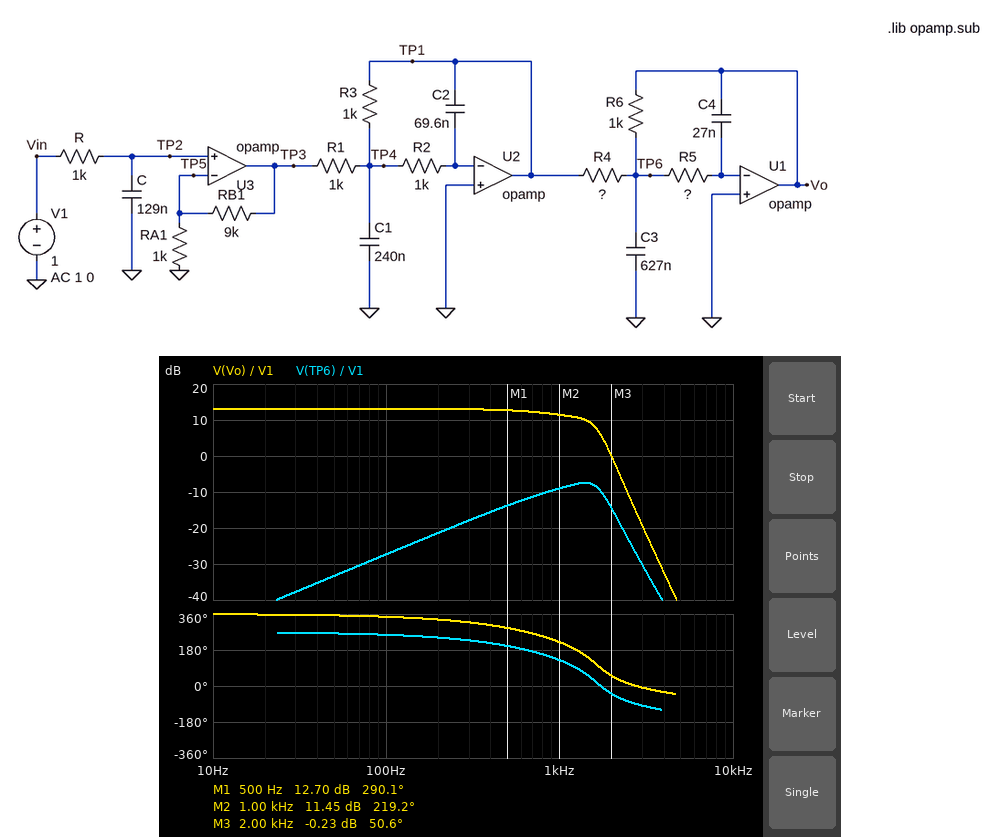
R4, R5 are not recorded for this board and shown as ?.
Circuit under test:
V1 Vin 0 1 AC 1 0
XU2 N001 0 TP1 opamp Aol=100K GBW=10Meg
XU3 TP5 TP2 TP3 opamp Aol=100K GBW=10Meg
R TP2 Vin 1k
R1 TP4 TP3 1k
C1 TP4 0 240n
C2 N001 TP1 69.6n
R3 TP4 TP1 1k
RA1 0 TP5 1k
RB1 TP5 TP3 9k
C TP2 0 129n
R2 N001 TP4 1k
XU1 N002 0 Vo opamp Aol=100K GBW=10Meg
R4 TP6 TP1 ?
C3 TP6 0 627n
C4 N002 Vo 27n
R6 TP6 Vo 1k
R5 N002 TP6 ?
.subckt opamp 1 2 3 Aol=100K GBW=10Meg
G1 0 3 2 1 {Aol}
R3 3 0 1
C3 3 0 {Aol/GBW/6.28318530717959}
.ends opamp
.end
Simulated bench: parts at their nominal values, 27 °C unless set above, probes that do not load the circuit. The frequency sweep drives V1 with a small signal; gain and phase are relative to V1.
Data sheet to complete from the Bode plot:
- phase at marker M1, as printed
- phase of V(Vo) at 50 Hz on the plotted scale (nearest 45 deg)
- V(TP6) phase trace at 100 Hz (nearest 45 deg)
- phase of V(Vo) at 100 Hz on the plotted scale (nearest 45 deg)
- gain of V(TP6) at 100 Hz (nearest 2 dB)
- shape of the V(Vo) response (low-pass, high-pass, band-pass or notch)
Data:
290.1 deg
360 deg
270 deg
360 deg
-28 dB
low-pass
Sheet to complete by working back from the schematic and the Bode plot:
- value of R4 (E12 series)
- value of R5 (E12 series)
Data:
2.2 kΩ
560 Ω
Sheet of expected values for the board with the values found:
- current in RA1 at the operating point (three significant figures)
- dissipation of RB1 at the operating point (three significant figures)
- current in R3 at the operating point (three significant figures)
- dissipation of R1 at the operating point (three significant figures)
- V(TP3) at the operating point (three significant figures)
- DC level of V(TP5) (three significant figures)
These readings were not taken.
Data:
1.00 mA
9.00 mW
10.0 mA
100 mW
10.0 V
1.00 V
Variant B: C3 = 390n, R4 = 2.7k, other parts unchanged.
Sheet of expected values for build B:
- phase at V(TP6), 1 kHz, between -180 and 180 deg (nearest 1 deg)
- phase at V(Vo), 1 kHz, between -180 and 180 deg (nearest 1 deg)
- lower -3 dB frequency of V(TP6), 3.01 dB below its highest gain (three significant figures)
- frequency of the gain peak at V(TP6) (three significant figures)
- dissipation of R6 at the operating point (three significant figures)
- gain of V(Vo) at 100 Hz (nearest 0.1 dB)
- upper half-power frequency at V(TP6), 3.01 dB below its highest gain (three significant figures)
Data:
134 deg
-136 deg
579 Hz
1.32 kHz
13.7 mW
11.3 dB
2.08 kHz
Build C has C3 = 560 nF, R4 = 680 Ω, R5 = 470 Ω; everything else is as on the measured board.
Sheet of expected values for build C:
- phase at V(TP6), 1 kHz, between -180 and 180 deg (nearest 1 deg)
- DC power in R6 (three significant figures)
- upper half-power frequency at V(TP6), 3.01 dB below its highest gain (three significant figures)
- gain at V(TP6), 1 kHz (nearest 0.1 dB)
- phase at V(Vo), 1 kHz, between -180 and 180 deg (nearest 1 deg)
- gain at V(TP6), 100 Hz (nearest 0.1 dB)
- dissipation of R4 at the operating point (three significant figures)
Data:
128 deg
216 mW
1.90 kHz
-1.6 dB
-142 deg
-18.6 dB
147 mW
